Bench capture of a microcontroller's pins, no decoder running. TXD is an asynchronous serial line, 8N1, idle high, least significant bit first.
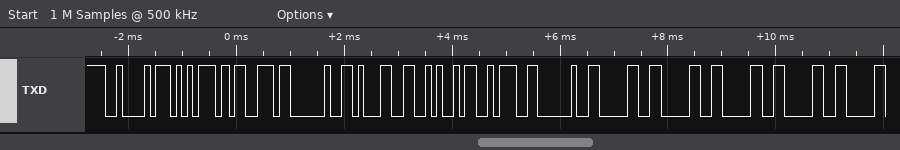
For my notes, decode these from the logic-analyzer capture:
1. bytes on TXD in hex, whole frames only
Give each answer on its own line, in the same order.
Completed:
0x42 0x75 0x73 0x20 0x31 0x4A 0x3A 0x20 0x30 0x30 0x30 0x30
